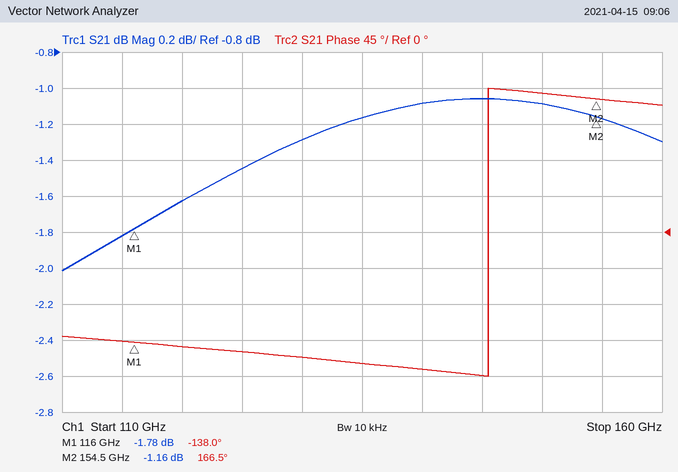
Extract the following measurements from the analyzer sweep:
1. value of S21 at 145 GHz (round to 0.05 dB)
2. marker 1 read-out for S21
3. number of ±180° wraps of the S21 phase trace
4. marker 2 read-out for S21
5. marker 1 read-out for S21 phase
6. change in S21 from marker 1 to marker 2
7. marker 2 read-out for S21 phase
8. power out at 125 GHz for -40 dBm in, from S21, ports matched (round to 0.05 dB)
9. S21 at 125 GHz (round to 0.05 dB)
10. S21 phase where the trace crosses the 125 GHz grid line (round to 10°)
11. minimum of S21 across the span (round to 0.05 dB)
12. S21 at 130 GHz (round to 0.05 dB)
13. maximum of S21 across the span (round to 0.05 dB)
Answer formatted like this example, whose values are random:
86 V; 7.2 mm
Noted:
-1.05 dB; -1.78 dB; 1; -1.16 dB; -138.0°; 0.62 dB; 166.5°; -41.45 dBm; -1.45 dB; -150°; -2.00 dB; -1.30 dB; -1.05 dB
